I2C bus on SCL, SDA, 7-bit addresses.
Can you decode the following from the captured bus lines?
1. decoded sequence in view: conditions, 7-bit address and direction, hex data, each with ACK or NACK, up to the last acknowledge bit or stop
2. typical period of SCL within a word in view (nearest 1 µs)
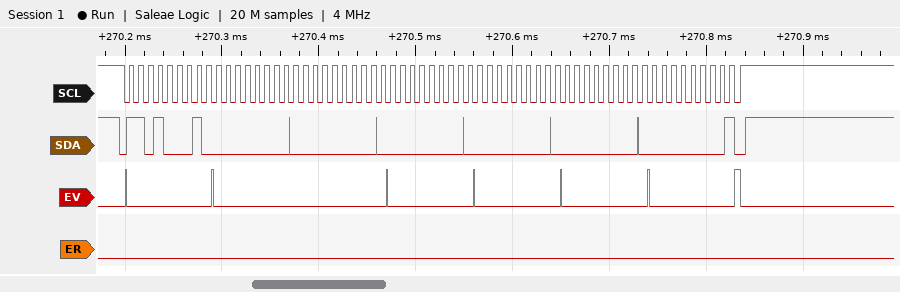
start, address 68 read ACK, 00 ACK, 00 ACK, 00 ACK, 00 ACK, 00 ACK, 00 NACK, stop
10 µs
